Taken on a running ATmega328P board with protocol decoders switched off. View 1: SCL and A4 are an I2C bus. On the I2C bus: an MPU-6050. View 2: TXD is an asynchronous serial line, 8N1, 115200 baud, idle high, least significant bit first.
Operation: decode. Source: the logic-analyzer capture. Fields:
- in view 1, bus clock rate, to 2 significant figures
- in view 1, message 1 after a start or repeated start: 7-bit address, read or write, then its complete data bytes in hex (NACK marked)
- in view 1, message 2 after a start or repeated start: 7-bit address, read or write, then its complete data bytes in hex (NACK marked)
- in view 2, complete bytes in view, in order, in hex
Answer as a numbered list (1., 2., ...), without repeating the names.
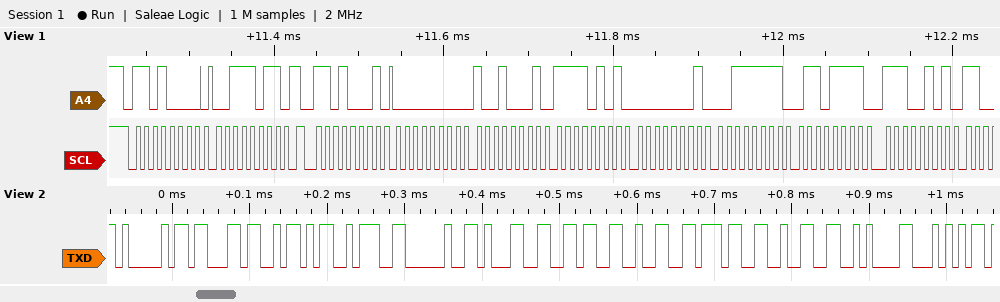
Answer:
1. 100 kHz
2. 0x68 write: 3B
3. 0x68 read: 00 91 F5 01 3F 6F E5
4. 0x41 0x63 0x5A 0x3A 0x20 0x31 0x36 0x32 0x37 0x32 0x0A 0x54
